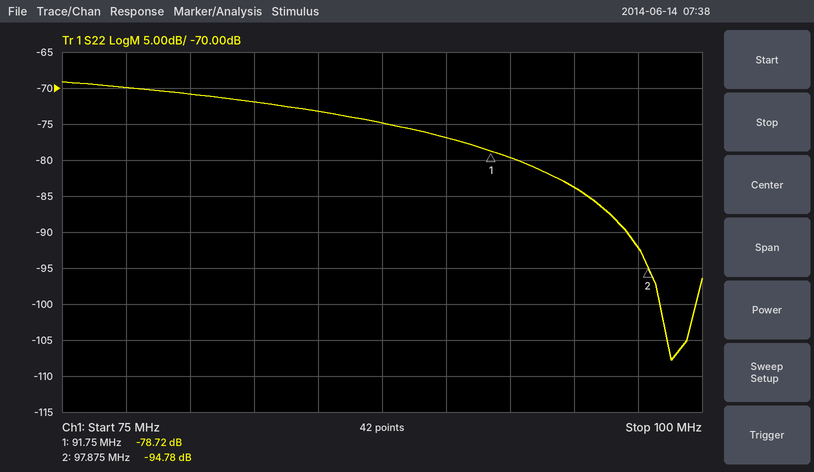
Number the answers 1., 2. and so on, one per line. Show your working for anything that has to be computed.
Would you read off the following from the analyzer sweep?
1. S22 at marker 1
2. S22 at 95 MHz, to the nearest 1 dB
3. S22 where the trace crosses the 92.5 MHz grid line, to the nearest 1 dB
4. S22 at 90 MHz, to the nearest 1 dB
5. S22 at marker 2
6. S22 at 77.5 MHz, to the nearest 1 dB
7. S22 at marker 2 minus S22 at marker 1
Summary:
1. -78.72 dB
2. -84 dB
3. -80 dB
4. -77 dB
5. -94.78 dB
6. -70 dB
7. -94.78 − (-78.72) = -16.06 dB
